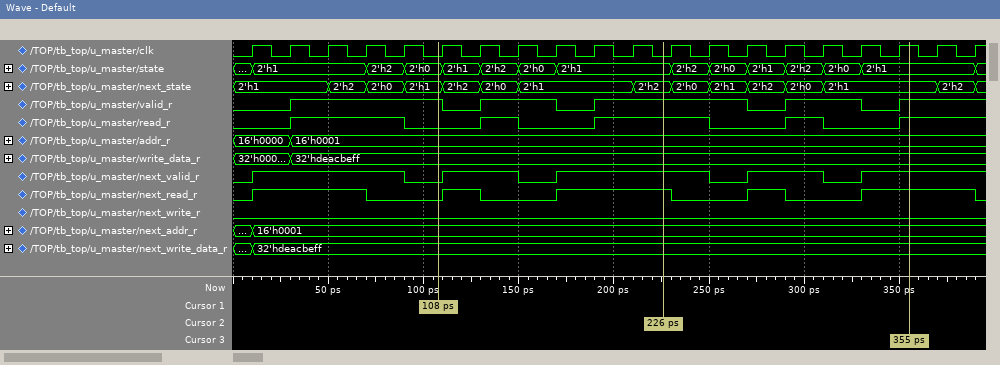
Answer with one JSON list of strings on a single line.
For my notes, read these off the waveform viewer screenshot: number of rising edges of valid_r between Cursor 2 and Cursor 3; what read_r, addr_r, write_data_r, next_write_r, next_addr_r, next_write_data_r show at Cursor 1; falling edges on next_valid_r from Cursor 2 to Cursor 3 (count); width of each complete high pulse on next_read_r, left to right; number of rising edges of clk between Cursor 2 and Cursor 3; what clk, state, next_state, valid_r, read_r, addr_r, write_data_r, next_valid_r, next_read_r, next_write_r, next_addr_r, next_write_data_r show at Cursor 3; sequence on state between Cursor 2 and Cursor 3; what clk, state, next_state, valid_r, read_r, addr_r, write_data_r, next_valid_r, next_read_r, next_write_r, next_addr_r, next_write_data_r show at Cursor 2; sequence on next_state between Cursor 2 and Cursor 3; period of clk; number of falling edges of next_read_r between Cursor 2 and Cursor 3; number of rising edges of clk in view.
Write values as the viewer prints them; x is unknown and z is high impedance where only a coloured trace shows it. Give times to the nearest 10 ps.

["2", "read_r=0, addr_r=16'h0001, write_data_r=32'hdeacbeff, next_write_r=0, next_addr_r=16'h0001, next_write_data_r=32'hdeacbeff", "2", "60 ps, 20 ps, 60 ps, 20 ps, 60 ps", "7", "clk=1, state=2'h1, next_state=2'h1, valid_r=1, read_r=1, addr_r=16'h0001, write_data_r=32'hdeacbeff, next_valid_r=1, next_read_r=1, next_write_r=0, next_addr_r=16'h0001, next_write_data_r=32'hdeacbeff", "2'h1, 2'h2, 2'h0, 2'h1, 2'h2, 2'h0, 2'h1", "clk=0, state=2'h1, next_state=2'h2, valid_r=1, read_r=1, addr_r=16'h0001, write_data_r=32'hdeacbeff, next_valid_r=1, next_read_r=1, next_write_r=0, next_addr_r=16'h0001, next_write_data_r=32'hdeacbeff", "2'h2, 2'h0, 2'h1, 2'h2, 2'h0, 2'h1", "20 ps", "2", "20"]
